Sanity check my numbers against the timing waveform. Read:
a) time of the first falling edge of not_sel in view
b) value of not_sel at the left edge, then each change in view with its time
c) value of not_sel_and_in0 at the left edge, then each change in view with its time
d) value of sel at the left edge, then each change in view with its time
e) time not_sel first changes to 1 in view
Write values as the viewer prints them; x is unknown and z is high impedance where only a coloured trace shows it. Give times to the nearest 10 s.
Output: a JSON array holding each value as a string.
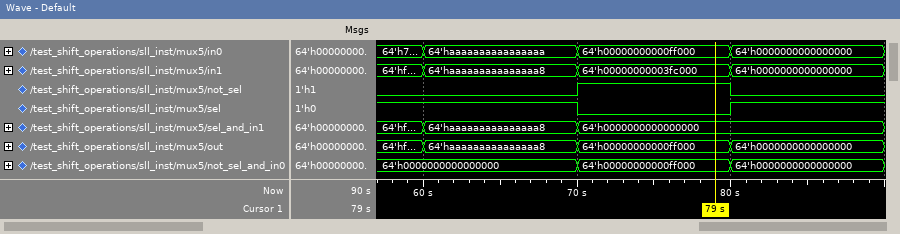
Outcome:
["80 s", "0, 1 at 70 s, 0 at 80 s", "64'h0000000000000000, 64'h00000000000ff000 at 70 s, 64'h0000000000000000 at 80 s", "1, 0 at 70 s, 1 at 80 s", "70 s"]
